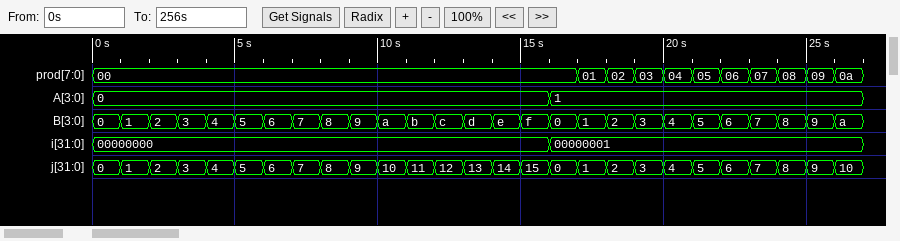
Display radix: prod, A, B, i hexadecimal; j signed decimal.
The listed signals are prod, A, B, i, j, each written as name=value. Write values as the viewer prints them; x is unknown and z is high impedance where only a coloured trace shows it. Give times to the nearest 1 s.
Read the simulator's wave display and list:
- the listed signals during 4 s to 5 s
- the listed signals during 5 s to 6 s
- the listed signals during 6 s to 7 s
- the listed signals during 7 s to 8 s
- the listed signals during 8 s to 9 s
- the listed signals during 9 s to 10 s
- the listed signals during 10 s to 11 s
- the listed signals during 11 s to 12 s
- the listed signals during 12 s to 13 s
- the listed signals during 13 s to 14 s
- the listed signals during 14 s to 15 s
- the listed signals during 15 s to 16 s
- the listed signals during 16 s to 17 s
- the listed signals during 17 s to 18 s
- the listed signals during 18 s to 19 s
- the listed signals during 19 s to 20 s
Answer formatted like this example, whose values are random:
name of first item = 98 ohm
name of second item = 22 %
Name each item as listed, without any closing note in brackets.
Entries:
the listed signals during 4 s to 5 s = prod=00, A=0, B=4, i=00000000, j=4
the listed signals during 5 s to 6 s = prod=00, A=0, B=5, i=00000000, j=5
the listed signals during 6 s to 7 s = prod=00, A=0, B=6, i=00000000, j=6
the listed signals during 7 s to 8 s = prod=00, A=0, B=7, i=00000000, j=7
the listed signals during 8 s to 9 s = prod=00, A=0, B=8, i=00000000, j=8
the listed signals during 9 s to 10 s = prod=00, A=0, B=9, i=00000000, j=9
the listed signals during 10 s to 11 s = prod=00, A=0, B=a, i=00000000, j=10
the listed signals during 11 s to 12 s = prod=00, A=0, B=b, i=00000000, j=11
the listed signals during 12 s to 13 s = prod=00, A=0, B=c, i=00000000, j=12
the listed signals during 13 s to 14 s = prod=00, A=0, B=d, i=00000000, j=13
the listed signals during 14 s to 15 s = prod=00, A=0, B=e, i=00000000, j=14
the listed signals during 15 s to 16 s = prod=00, A=0, B=f, i=00000000, j=15
the listed signals during 16 s to 17 s = prod=00, A=1, B=0, i=00000001, j=0
the listed signals during 17 s to 18 s = prod=01, A=1, B=1, i=00000001, j=1
the listed signals during 18 s to 19 s = prod=02, A=1, B=2, i=00000001, j=2
the listed signals during 19 s to 20 s = prod=03, A=1, B=3, i=00000001, j=3
